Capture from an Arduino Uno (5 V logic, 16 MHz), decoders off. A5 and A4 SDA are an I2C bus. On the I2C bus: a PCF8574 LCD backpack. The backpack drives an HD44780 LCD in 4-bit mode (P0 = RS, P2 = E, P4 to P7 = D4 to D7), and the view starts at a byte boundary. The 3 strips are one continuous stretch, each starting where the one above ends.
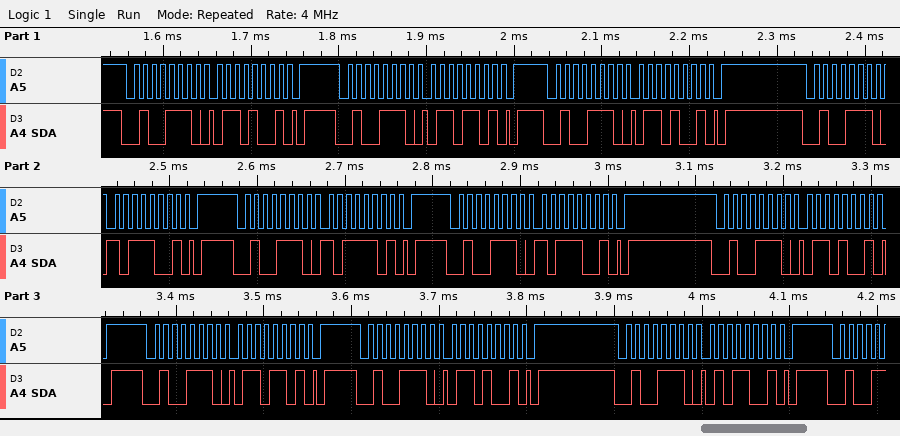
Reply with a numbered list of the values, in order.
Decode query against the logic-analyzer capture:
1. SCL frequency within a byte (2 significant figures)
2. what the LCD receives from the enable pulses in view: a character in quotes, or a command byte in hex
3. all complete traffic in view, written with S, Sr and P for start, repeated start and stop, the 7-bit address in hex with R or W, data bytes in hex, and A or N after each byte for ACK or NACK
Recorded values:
1. 100 kHz
2. 'k'
3. S 27W A 69 A P S 27W A 6D A P S 27W A 69 A P S 27W A B9 A P S 27W A BD A P S 27W A B9 A P S 27W A 69 A P S 27W A 6D A P S 27W A 69 A P S 27W A 59 A P
